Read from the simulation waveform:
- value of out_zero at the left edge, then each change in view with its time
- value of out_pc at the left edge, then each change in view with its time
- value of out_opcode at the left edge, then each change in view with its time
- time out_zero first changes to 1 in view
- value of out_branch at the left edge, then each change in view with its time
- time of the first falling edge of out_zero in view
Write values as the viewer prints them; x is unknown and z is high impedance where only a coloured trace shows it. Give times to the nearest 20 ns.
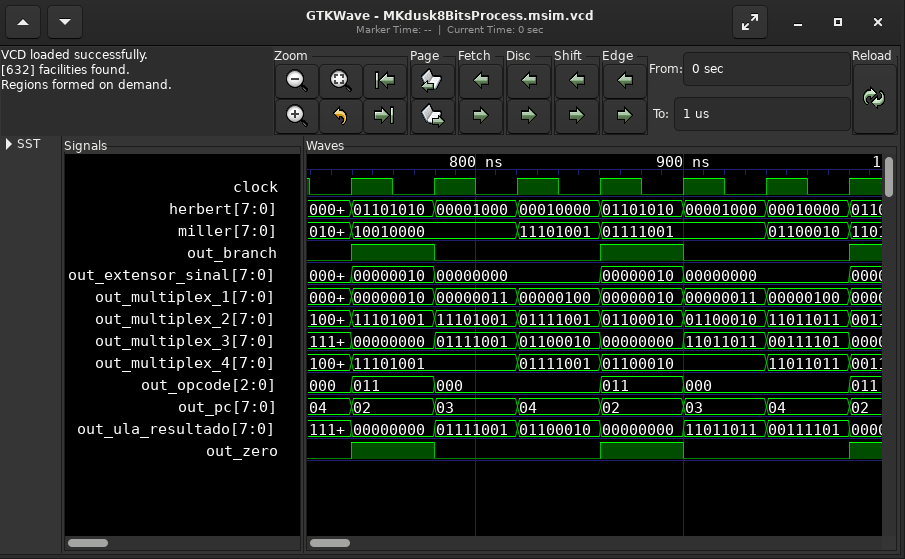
0, 1 at 740 ns, 0 at 780 ns, 1 at 860 ns, 0 at 900 ns, 1 at 980 ns
04, 02 at 740 ns, 03 at 780 ns, 04 at 820 ns, 02 at 860 ns, 03 at 900 ns, 04 at 940 ns, 02 at 980 ns
000, 011 at 740 ns, 000 at 780 ns, 011 at 860 ns, 000 at 900 ns, 011 at 980 ns
740 ns
0, 1 at 740 ns, 0 at 780 ns, 1 at 860 ns, 0 at 900 ns, 1 at 980 ns
780 ns
